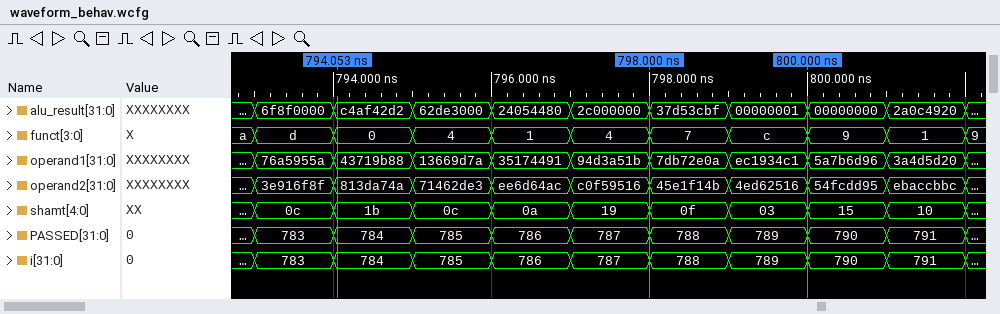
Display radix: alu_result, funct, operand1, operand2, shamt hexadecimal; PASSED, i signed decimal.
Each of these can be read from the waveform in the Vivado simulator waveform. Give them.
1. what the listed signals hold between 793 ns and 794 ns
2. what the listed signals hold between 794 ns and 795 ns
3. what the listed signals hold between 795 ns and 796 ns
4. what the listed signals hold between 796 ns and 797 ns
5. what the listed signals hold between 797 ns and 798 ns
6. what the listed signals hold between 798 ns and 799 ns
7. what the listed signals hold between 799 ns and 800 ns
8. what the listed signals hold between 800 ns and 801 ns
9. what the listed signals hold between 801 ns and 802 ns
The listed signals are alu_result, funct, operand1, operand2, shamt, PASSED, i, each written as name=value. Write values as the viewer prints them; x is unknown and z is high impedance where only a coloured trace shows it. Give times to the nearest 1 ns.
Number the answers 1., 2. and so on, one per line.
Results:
1. alu_result=6f8f0000, funct=d, operand1=76a5955a, operand2=3e916f8f, shamt=0c, PASSED=783, i=783
2. alu_result=c4af42d2, funct=0, operand1=43719b88, operand2=813da74a, shamt=1b, PASSED=784, i=784
3. alu_result=62de3000, funct=4, operand1=13669d7a, operand2=71462de3, shamt=0c, PASSED=785, i=785
4. alu_result=24054480, funct=1, operand1=35174491, operand2=ee6d64ac, shamt=0a, PASSED=786, i=786
5. alu_result=2c000000, funct=4, operand1=94d3a51b, operand2=c0f59516, shamt=19, PASSED=787, i=787
6. alu_result=37d53cbf, funct=7, operand1=7db72e0a, operand2=45e1f14b, shamt=0f, PASSED=788, i=788
7. alu_result=00000001, funct=c, operand1=ec1934c1, operand2=4ed62516, shamt=03, PASSED=789, i=789
8. alu_result=00000000, funct=9, operand1=5a7b6d96, operand2=54fcdd95, shamt=15, PASSED=790, i=790
9. alu_result=2a0c4920, funct=1, operand1=3a4d5d20, operand2=ebaccbbc, shamt=10, PASSED=791, i=791
